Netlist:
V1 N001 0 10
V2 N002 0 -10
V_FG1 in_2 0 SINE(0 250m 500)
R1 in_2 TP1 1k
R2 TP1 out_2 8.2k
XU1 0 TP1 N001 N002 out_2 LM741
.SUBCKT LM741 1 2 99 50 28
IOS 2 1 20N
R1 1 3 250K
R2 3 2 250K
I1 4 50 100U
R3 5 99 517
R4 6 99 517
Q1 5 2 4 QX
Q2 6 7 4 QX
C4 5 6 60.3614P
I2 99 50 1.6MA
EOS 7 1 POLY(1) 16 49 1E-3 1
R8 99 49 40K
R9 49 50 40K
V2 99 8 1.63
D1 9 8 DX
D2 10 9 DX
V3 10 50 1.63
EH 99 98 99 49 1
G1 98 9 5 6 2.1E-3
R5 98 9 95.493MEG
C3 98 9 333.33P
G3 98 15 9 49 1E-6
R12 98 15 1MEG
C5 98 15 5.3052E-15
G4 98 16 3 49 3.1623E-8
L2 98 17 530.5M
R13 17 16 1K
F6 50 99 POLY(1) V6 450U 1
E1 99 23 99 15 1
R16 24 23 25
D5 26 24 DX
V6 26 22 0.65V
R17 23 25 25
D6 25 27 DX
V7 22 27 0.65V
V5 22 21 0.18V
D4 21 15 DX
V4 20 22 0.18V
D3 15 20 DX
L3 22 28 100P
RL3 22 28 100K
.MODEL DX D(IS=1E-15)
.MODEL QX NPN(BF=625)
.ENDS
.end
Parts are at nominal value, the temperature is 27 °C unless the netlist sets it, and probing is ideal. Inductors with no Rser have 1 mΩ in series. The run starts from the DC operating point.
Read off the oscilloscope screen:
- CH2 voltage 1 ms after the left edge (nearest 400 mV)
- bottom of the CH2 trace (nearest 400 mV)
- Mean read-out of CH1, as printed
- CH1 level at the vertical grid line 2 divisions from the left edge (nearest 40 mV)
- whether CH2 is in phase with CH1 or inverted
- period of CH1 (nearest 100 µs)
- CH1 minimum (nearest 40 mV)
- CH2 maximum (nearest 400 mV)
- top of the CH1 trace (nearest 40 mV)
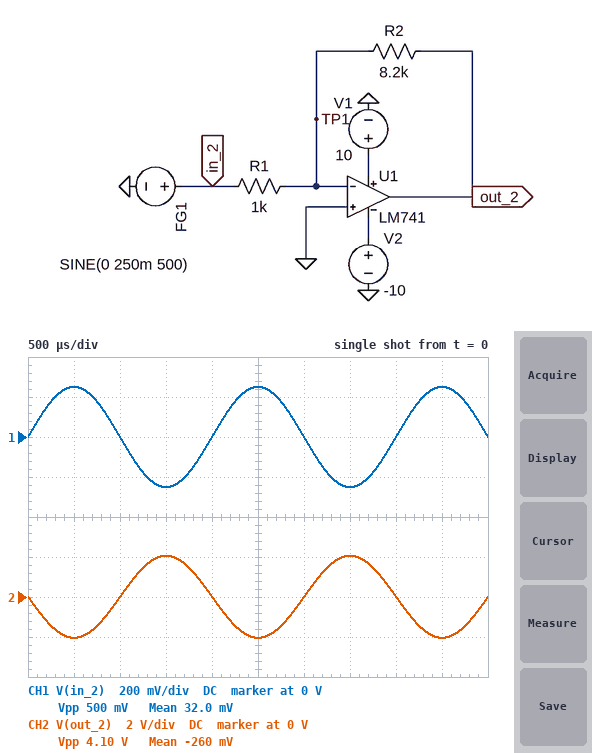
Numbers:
0 V
-2.0 V
32.0 mV
0 V
inverted
2.0 ms
-240 mV
2.0 V
240 mV
